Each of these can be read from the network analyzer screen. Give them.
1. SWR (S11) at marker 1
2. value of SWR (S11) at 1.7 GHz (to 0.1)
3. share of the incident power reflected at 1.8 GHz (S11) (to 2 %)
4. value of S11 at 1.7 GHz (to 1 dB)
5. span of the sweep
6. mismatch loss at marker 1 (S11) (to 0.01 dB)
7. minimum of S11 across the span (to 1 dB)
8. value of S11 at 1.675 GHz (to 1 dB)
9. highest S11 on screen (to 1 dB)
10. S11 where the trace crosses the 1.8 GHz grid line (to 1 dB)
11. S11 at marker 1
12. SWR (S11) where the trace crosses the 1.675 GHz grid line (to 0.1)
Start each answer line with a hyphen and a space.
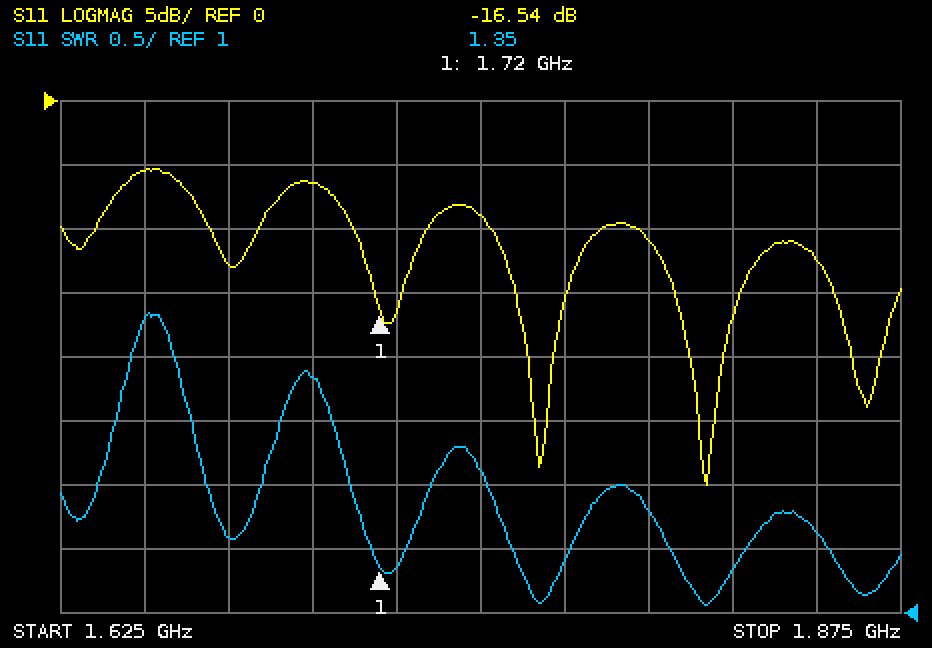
- 1.35
- 2.8
- 8 %
- -6 dB
- 250 MHz
- 0.10 dB
- -30 dB
- -13 dB
- -5 dB
- -11 dB
- -16.54 dB
- 1.6
